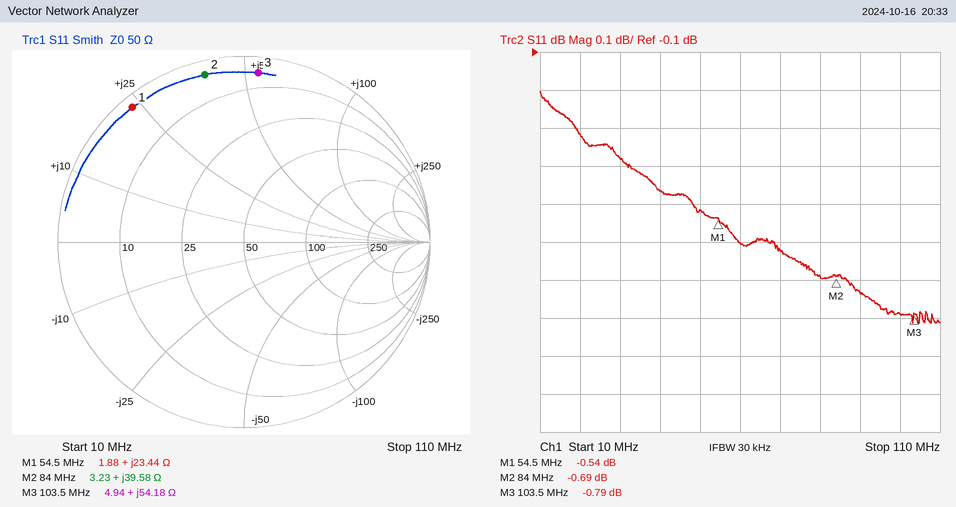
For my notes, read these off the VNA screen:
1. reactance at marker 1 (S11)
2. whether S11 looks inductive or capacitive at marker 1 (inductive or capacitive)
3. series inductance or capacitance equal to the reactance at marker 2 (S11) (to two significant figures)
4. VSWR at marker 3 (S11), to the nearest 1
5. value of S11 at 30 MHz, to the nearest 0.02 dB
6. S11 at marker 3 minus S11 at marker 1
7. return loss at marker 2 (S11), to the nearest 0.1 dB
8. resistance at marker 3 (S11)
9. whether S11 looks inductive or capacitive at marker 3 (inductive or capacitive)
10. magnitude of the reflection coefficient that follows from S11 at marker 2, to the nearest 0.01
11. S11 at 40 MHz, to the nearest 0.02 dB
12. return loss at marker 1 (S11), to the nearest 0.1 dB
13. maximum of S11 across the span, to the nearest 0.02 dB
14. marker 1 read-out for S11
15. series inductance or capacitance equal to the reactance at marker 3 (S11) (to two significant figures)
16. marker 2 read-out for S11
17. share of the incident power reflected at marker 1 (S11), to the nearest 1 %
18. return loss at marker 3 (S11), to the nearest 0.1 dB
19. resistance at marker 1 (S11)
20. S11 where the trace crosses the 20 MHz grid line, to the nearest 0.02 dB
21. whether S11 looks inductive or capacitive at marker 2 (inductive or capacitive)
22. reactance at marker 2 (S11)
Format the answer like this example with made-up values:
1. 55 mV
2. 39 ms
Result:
1. +23.44 Ω
2. inductive
3. 75 nH
4. 22
5. -0.38 dB
6. -0.25 dB
7. 0.7 dB
8. 4.94 Ω
9. inductive
10. 0.92
11. -0.46 dB
12. 0.5 dB
13. -0.20 dB
14. -0.54 dB
15. 83 nH
16. -0.69 dB
17. 88 %
18. 0.8 dB
19. 1.88 Ω
20. -0.32 dB
21. inductive
22. +39.58 Ω
